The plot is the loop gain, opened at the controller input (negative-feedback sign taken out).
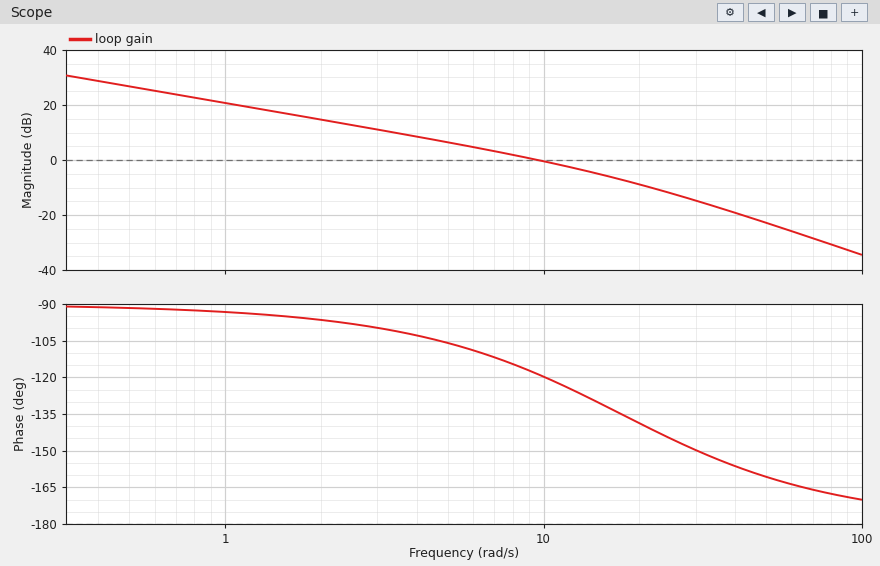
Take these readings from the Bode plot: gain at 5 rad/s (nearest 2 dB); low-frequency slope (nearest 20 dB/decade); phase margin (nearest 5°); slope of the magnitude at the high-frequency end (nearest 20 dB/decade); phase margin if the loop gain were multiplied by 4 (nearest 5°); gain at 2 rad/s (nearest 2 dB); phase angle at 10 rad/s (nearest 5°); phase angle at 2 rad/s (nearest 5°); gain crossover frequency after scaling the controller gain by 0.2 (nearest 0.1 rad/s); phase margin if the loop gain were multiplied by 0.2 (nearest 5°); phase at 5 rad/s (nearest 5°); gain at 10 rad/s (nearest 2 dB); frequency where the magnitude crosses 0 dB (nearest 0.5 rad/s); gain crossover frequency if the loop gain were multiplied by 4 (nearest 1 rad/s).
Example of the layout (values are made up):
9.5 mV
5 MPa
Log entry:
6 dB
-20 dB/decade
60°
-40 dB/decade
35°
14 dB
-120°
-95°
2.2 rad/s
85°
-105°
0 dB
9.5 rad/s
25 rad/s
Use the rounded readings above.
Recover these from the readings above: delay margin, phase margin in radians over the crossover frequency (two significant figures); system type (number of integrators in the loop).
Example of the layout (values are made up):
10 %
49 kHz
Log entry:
0.11 s
1
